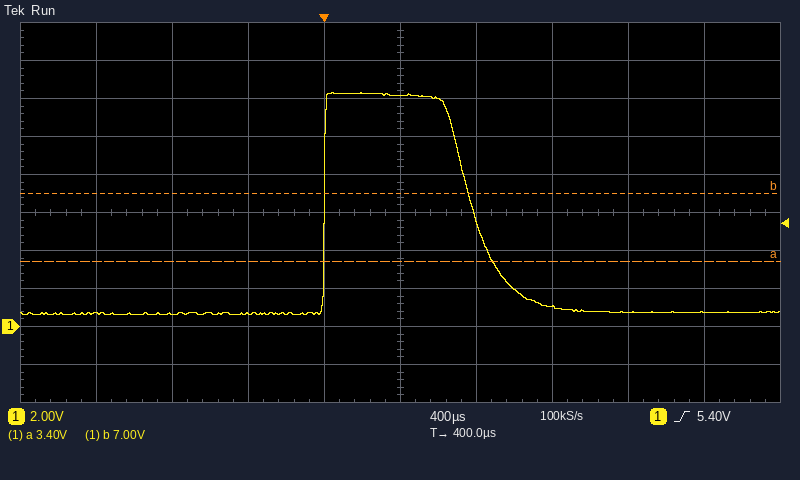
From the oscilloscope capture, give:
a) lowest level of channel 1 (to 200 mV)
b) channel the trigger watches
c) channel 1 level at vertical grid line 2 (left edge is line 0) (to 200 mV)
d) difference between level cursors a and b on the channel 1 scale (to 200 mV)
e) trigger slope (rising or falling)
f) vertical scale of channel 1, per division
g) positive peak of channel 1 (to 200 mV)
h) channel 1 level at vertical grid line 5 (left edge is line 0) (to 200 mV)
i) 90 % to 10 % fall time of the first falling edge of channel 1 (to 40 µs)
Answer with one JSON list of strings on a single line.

["600 mV", "channel 1", "600 mV", "3.6 V", "rising", "2 V", "12.4 V", "12.2 V", "360 µs"]
